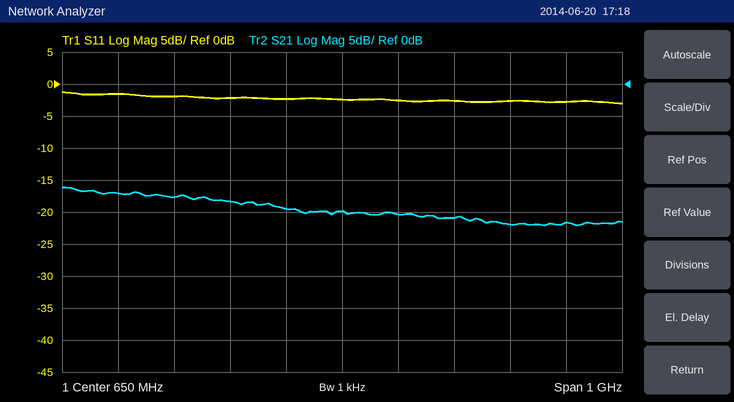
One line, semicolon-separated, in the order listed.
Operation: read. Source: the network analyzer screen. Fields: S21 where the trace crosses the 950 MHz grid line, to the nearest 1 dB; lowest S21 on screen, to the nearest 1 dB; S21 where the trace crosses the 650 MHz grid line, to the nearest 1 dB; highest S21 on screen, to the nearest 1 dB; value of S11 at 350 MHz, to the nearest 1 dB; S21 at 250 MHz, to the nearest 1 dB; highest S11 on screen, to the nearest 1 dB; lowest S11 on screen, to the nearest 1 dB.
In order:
-22 dB; -22 dB; -20 dB; -16 dB; -2 dB; -17 dB; -1 dB; -3 dB
